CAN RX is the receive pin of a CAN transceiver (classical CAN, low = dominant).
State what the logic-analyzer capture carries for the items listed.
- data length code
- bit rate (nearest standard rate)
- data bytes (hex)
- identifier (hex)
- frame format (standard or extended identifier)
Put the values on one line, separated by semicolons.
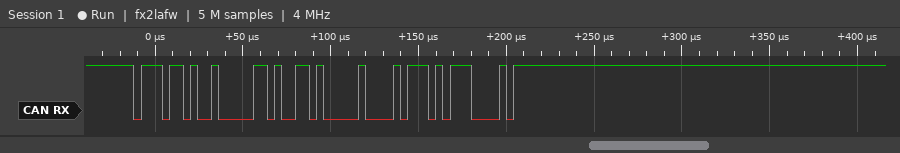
2; 250 kbit/s; 9A 00; 0x769; standard
